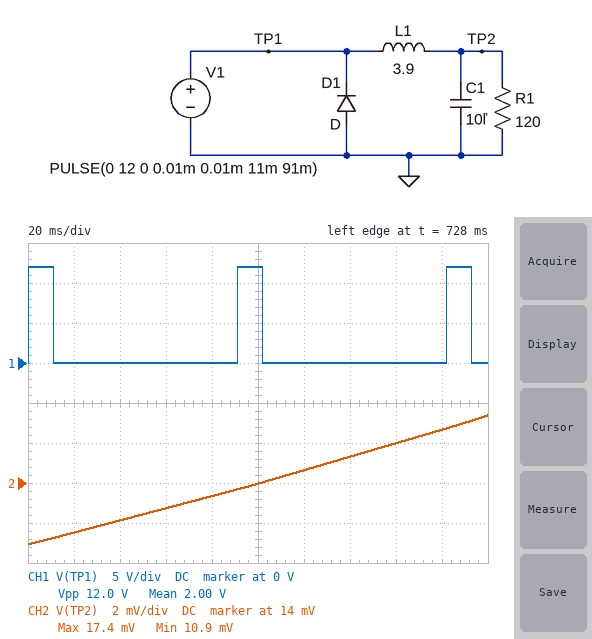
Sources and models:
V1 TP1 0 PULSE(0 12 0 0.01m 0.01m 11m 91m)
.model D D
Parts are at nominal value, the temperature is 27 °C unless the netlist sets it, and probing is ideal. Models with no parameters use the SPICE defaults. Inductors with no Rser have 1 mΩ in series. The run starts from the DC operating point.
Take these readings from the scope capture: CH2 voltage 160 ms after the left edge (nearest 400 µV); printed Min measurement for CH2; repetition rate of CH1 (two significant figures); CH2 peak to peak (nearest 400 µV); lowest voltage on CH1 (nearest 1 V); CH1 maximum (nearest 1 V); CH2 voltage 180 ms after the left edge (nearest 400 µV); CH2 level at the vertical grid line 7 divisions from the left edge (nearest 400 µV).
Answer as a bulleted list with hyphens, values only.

- 16.0 mV
- 10.9 mV
- 11 Hz
- 6.4 mV
- 0 V
- 12 V
- 16.8 mV
- 15.2 mV
